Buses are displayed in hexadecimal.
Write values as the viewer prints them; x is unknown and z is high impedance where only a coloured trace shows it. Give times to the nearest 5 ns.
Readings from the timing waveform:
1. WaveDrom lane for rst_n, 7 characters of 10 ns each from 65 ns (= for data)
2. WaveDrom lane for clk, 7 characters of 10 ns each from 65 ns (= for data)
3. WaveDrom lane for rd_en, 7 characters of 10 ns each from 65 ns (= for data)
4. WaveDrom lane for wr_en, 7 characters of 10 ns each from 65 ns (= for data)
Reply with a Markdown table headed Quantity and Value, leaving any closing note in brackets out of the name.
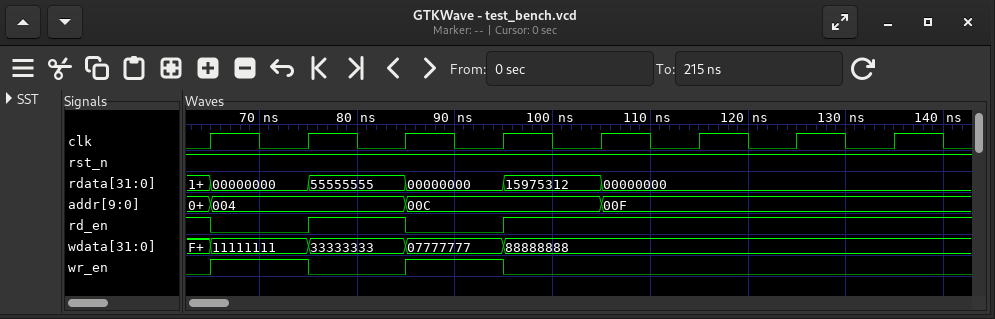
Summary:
| Quantity | Value |
|---|---|
| WaveDrom lane for rst_n, 7 characters of 10 ns each from 65 ns | {name: 'rst_n', wave: '1......'} |
| WaveDrom lane for clk, 7 characters of 10 ns each from 65 ns | {name: 'clk', wave: 'p......'} |
| WaveDrom lane for rd_en, 7 characters of 10 ns each from 65 ns | {name: 'rd_en', wave: '0101...'} |
| WaveDrom lane for wr_en, 7 characters of 10 ns each from 65 ns | {name: 'wr_en', wave: '1010...'} |
